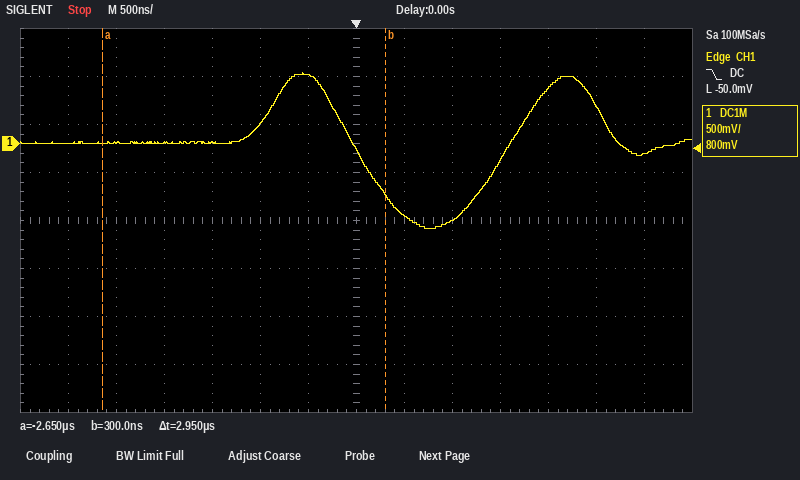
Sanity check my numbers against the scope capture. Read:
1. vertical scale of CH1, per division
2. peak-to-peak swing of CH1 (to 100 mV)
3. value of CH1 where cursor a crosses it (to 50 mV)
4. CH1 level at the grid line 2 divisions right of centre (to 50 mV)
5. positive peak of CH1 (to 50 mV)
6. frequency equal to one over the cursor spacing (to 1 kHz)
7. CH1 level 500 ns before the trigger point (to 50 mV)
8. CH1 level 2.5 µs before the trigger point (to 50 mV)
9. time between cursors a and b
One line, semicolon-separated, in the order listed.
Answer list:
500 mV; 1.60 V; 0 mV; -800 mV; 750 mV; 339 kHz; 700 mV; 0 mV; 2.95 µs
